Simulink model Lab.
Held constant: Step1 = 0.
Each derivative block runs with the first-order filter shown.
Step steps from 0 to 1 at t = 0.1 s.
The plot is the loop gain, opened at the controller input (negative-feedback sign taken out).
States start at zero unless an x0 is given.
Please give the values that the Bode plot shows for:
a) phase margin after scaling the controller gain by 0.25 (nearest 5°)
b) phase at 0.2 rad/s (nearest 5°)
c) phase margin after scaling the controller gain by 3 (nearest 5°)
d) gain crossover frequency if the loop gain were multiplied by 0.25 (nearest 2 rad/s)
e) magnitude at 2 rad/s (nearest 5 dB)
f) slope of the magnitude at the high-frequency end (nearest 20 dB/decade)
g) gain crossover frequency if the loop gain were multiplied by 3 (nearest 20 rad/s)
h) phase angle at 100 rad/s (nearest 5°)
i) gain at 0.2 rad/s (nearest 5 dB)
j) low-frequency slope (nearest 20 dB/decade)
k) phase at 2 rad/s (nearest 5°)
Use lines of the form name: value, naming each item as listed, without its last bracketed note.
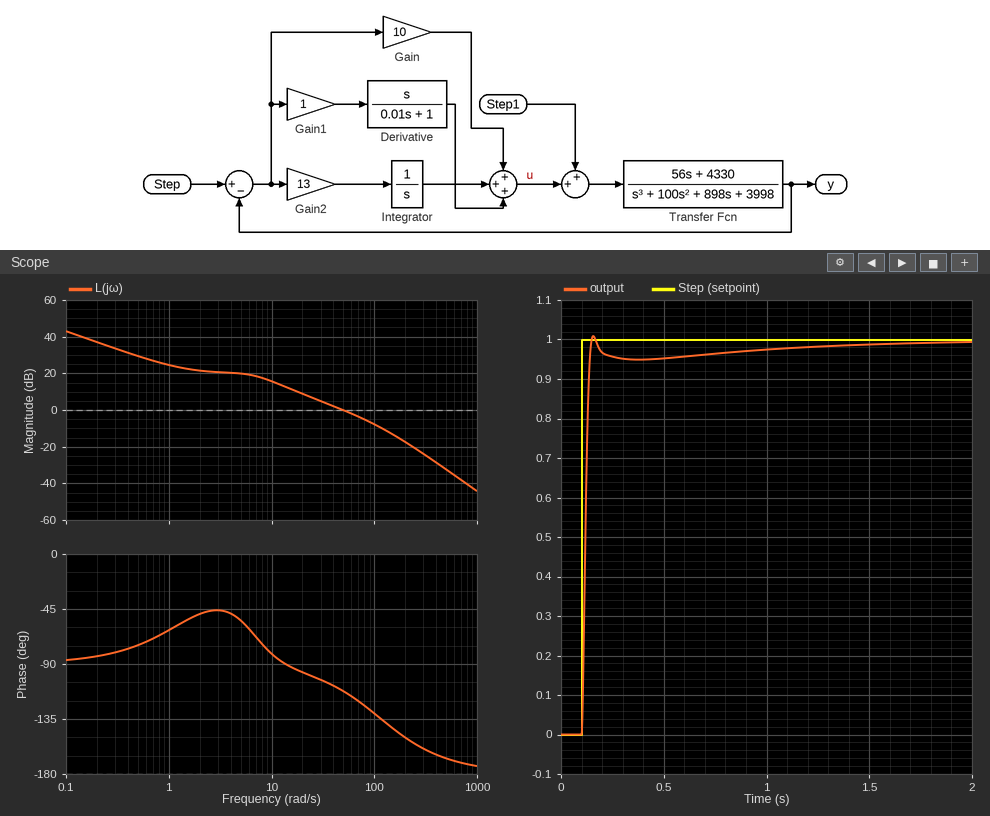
phase margin after scaling the controller gain by 0.25: 90°
phase at 0.2 rad/s: -85°
phase margin after scaling the controller gain by 3: 45°
gain crossover frequency if the loop gain were multiplied by 0.25: 14 rad/s
magnitude at 2 rad/s: 20 dB
slope of the magnitude at the high-frequency end: -40 dB/decade
gain crossover frequency if the loop gain were multiplied by 3: 120 rad/s
phase angle at 100 rad/s: -130°
gain at 0.2 rad/s: 35 dB
low-frequency slope: -20 dB/decade
phase at 2 rad/s: -50°
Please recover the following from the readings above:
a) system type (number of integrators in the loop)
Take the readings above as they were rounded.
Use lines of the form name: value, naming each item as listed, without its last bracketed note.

system type: 1
